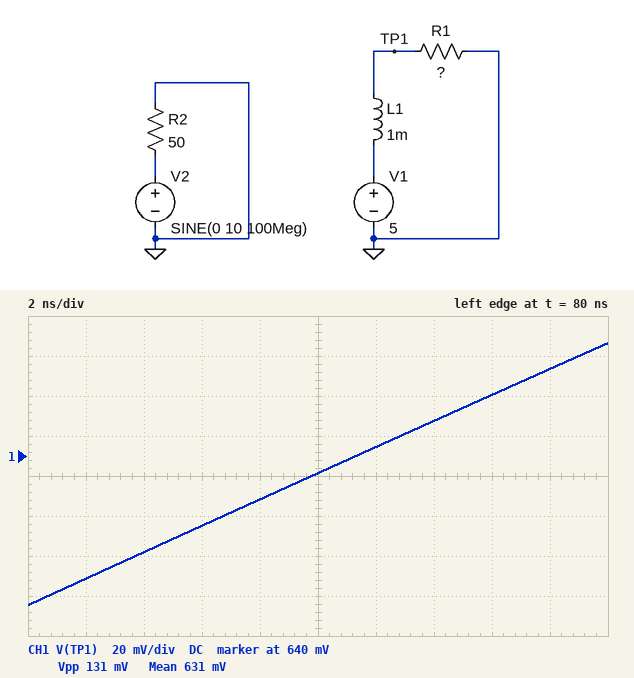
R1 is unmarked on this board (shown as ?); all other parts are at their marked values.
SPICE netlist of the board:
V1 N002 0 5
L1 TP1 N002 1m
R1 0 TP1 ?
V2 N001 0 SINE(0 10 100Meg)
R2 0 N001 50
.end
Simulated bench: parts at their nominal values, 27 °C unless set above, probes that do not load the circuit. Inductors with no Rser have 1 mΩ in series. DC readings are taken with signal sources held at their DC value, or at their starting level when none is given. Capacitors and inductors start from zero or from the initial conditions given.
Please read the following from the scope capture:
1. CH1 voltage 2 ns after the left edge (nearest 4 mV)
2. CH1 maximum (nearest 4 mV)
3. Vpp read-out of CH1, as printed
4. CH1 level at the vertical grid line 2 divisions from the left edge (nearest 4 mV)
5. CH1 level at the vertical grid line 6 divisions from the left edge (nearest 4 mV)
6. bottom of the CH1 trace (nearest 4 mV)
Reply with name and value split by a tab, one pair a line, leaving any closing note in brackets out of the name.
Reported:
CH1 voltage 2 ns after the left edge	580 mV
CH1 maximum	696 mV
Vpp read-out of CH1, as printed	131 mV
CH1 level at the vertical grid line 2 divisions from the left edge	592 mV
CH1 level at the vertical grid line 6 divisions from the left edge	644 mV
bottom of the CH1 trace	564 mV
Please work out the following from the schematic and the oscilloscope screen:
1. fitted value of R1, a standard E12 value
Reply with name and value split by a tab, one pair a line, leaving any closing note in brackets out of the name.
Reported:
fitted value of R1, a standard E12 value	1.5 kΩ
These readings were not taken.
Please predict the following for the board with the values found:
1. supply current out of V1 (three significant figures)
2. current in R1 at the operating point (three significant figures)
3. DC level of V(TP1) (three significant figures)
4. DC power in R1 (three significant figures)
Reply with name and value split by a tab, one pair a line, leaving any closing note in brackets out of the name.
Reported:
supply current out of V1	3.33 mA
current in R1 at the operating point	3.33 mA
DC level of V(TP1)	5.00 V
DC power in R1	16.7 mW
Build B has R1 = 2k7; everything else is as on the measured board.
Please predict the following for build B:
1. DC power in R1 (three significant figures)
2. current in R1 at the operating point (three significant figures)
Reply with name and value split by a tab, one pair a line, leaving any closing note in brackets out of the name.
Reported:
DC power in R1	9.26 mW
current in R1 at the operating point	1.85 mA
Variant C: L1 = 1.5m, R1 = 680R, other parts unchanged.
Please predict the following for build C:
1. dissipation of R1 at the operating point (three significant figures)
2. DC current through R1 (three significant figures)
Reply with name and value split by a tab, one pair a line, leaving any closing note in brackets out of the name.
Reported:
dissipation of R1 at the operating point	36.8 mW
DC current through R1	7.35 mA
